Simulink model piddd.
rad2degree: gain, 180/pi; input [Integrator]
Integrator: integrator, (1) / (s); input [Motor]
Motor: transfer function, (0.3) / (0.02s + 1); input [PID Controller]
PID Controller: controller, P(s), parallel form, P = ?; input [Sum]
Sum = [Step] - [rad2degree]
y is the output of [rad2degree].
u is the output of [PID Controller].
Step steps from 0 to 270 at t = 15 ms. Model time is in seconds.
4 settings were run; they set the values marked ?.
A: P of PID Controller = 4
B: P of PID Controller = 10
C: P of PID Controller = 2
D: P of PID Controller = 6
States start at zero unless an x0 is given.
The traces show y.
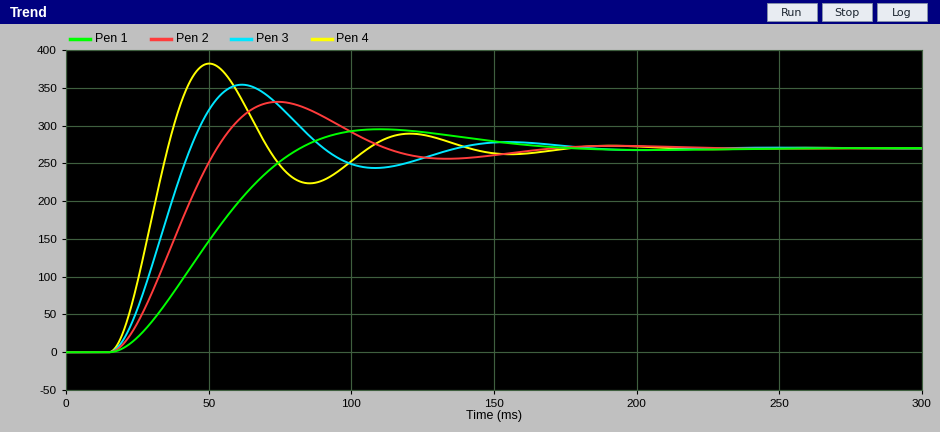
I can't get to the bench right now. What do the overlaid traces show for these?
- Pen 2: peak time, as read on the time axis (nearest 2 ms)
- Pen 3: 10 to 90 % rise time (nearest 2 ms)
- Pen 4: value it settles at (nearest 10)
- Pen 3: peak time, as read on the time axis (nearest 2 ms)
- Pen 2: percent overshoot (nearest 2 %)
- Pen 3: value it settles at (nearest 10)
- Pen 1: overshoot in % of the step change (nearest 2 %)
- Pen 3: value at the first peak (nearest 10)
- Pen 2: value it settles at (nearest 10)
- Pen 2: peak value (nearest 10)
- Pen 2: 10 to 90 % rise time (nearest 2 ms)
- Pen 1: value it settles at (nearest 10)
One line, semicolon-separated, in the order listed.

74 ms; 20 ms; 270; 62 ms; 22 %; 270; 10 %; 350; 270; 330; 26 ms; 270
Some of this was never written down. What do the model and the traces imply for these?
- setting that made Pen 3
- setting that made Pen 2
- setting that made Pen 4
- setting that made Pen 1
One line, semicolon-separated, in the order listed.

D; A; B; C
